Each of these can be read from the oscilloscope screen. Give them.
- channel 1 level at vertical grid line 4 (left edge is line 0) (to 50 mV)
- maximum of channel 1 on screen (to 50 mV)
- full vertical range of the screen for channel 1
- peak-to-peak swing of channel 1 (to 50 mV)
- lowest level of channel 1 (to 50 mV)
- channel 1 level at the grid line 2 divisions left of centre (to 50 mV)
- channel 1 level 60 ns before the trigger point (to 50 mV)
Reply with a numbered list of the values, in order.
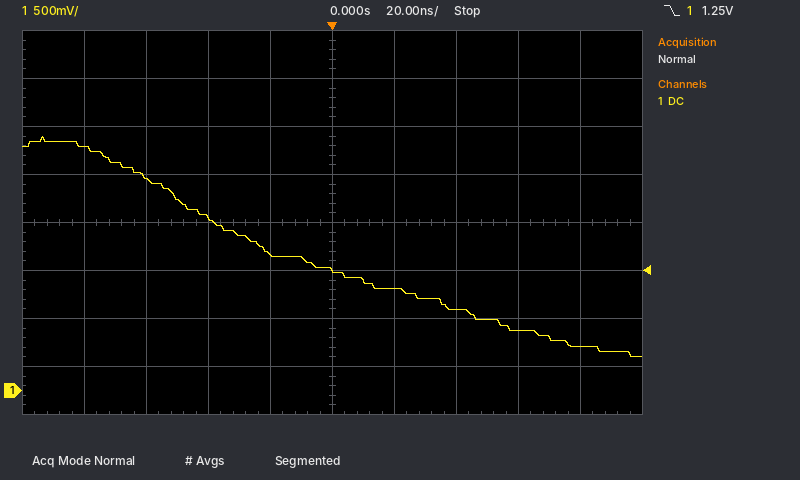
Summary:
1. 1.40 V
2. 2.65 V
3. 4 V
4. 2.30 V
5. 350 mV
6. 1.80 V
7. 2.20 V
